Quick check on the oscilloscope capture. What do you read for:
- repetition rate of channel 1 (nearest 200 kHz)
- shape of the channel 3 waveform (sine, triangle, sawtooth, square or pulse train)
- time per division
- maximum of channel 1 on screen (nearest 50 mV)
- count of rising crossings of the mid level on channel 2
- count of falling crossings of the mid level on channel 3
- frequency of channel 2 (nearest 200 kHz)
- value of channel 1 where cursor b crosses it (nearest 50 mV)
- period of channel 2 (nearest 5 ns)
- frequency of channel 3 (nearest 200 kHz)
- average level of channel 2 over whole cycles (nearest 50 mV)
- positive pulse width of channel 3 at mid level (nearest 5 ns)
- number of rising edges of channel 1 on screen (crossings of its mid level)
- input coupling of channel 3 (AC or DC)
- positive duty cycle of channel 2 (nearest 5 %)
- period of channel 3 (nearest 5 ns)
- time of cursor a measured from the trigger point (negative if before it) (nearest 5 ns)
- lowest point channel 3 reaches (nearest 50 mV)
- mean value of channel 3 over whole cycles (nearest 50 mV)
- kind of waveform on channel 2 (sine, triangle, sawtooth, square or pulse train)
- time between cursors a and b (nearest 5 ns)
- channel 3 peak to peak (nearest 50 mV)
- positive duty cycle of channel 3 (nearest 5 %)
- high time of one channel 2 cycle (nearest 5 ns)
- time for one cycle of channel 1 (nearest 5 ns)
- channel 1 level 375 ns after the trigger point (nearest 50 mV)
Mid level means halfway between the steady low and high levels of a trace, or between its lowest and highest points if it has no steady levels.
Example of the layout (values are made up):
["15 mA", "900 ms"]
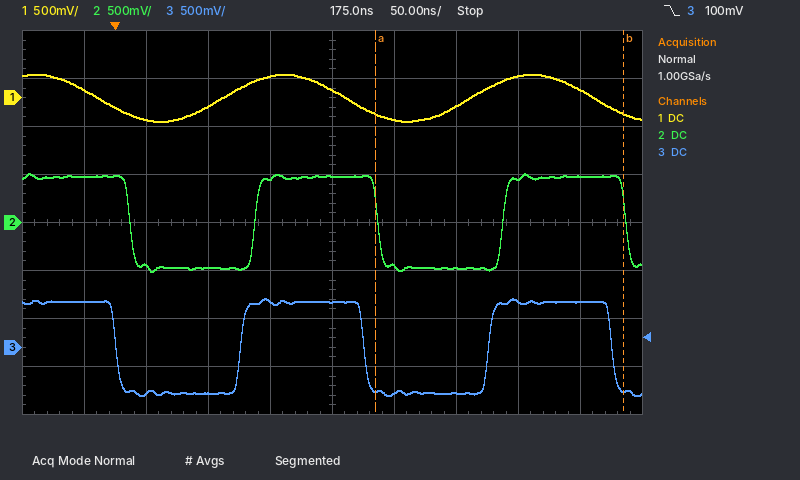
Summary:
["5.0 MHz", "square", "50 ns", "250 mV", "2", "3", "5.0 MHz", "-150 mV", "200 ns", "5.0 MHz", "0 mV", "100 ns", "2", "DC", "50 %", "200 ns", "+210 ns", "-500 mV", "0 mV", "square", "200 ns", "1.00 V", "50 %", "100 ns", "200 ns", "100 mV"]
